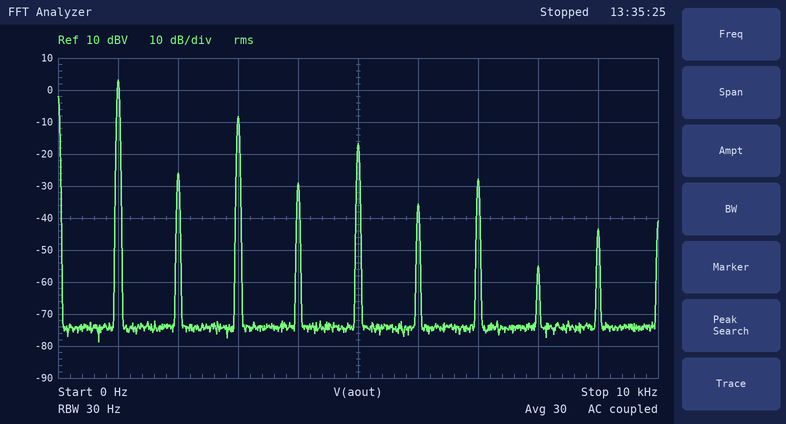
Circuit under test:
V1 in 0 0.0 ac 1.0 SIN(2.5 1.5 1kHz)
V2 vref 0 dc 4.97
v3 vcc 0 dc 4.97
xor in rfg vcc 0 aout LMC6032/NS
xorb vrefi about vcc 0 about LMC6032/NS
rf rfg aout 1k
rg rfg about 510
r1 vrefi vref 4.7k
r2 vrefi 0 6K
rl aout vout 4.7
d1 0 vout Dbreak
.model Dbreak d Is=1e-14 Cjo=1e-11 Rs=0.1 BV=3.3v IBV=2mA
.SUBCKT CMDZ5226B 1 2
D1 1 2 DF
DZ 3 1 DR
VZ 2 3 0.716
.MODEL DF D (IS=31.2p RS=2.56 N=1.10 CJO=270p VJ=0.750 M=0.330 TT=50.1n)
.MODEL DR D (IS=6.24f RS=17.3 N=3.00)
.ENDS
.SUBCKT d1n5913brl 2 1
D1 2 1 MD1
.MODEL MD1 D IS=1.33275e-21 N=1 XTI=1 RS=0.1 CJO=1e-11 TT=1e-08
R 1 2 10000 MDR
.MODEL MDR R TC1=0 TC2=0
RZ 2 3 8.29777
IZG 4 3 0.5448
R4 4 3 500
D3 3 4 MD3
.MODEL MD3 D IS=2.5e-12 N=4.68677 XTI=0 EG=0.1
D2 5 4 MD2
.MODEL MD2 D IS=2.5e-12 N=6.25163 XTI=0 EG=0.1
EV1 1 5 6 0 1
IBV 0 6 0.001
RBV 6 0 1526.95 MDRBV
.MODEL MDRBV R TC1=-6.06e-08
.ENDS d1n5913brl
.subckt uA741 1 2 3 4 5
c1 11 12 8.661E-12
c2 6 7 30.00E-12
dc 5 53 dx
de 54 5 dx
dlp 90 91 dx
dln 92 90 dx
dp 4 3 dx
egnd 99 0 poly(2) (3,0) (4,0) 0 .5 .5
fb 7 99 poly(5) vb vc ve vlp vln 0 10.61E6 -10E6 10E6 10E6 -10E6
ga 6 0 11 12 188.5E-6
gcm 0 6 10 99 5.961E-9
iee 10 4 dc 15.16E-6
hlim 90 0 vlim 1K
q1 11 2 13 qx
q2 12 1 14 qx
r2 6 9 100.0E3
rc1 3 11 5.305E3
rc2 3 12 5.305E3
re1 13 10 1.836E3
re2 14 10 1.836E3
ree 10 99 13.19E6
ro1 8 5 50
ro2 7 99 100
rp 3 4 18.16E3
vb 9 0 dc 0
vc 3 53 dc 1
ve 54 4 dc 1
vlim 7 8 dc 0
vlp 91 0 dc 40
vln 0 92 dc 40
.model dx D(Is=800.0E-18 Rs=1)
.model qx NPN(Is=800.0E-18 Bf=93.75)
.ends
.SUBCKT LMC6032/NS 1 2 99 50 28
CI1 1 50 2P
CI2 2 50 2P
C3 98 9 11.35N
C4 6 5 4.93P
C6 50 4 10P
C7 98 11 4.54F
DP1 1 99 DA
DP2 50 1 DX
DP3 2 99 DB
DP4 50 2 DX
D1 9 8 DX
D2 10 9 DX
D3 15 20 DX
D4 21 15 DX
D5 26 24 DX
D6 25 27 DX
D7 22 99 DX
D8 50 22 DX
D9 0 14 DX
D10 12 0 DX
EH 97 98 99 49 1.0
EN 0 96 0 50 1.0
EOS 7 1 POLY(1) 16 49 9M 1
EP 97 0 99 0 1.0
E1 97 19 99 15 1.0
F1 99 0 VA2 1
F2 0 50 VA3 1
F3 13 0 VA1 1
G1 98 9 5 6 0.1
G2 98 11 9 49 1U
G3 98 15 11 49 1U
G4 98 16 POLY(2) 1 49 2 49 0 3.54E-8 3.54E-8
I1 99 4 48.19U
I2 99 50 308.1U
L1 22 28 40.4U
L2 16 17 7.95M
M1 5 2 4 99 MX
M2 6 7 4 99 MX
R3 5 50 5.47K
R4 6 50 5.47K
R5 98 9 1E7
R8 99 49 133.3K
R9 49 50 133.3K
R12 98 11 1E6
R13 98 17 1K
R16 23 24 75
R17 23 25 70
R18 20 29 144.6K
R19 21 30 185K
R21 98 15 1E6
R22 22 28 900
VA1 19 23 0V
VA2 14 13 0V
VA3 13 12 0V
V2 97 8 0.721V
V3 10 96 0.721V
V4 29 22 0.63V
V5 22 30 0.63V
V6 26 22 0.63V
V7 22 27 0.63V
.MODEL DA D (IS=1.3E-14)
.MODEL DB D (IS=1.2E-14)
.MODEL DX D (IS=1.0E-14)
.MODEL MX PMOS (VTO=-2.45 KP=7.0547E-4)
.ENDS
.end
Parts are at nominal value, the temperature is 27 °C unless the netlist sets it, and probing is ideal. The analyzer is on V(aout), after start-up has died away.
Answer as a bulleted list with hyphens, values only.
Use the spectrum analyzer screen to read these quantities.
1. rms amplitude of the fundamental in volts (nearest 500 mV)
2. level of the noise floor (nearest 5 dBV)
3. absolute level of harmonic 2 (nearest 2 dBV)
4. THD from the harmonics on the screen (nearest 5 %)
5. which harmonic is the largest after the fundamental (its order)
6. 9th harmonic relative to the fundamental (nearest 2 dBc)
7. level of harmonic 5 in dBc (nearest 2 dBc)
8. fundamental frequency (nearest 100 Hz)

- 1.5 V
- -75 dBV
- -26 dBV
- 30 %
- 3
- -46 dBc
- -20 dBc
- 1.0 kHz
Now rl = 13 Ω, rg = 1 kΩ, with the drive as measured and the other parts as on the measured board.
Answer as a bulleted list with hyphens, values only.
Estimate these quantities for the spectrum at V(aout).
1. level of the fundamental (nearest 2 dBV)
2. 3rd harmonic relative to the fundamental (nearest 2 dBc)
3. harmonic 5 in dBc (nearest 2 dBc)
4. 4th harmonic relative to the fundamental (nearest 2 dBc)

- 2 dBV
- -14 dBc
- -32 dBc
- -26 dBc
